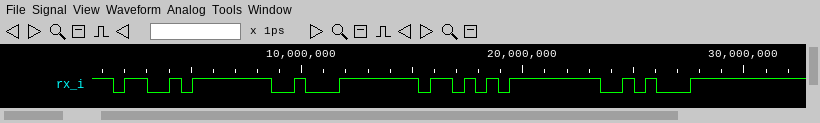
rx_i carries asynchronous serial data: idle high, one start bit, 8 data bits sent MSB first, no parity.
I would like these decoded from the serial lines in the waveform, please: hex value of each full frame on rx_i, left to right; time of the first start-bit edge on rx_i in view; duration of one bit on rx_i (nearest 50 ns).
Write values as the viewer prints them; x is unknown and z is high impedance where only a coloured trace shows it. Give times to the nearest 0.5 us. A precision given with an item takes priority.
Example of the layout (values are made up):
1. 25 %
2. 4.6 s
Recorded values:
1. CB, 47, D5, 51
2. 1.5 us
3. 500 ns
